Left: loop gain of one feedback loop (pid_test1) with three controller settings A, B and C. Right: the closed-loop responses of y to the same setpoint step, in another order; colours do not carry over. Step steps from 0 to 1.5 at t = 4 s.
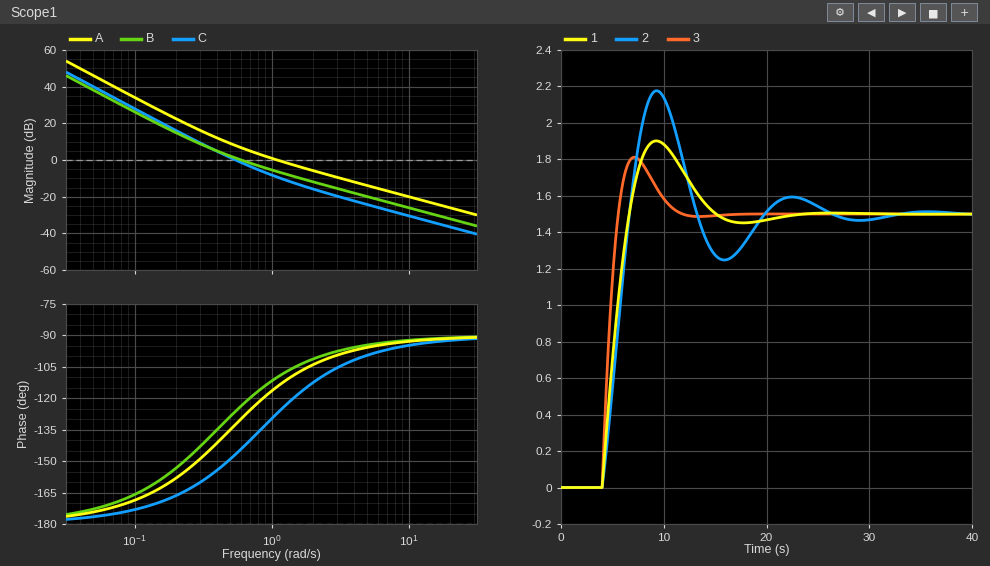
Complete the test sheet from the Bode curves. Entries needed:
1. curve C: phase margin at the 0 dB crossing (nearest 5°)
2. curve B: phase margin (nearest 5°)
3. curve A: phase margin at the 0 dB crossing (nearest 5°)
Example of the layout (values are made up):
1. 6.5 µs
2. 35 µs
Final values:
1. 35°
2. 55°
3. 65°
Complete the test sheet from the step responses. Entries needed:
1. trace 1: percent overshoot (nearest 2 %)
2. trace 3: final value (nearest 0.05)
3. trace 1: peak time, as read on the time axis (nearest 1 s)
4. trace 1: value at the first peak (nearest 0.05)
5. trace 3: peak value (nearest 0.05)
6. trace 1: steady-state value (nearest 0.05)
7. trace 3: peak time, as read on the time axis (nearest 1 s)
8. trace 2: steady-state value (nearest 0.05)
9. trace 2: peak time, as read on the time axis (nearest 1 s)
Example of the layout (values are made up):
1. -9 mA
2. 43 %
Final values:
1. 26 %
2. 1.50
3. 9 s
4. 1.90
5. 1.80
6. 1.50
7. 7 s
8. 1.50
9. 9 s
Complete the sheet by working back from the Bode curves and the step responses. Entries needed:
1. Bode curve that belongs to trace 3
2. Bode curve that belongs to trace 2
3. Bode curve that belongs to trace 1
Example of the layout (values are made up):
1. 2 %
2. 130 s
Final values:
1. A
2. C
3. B
